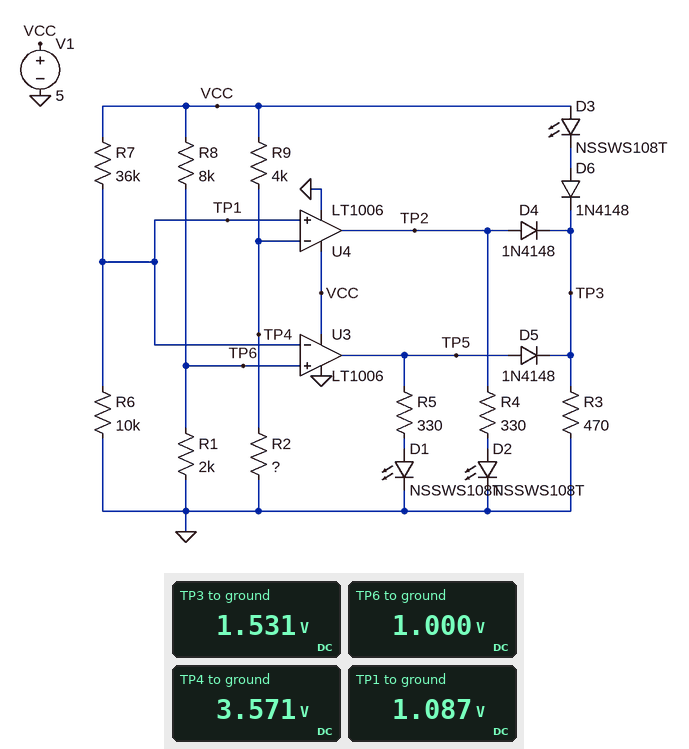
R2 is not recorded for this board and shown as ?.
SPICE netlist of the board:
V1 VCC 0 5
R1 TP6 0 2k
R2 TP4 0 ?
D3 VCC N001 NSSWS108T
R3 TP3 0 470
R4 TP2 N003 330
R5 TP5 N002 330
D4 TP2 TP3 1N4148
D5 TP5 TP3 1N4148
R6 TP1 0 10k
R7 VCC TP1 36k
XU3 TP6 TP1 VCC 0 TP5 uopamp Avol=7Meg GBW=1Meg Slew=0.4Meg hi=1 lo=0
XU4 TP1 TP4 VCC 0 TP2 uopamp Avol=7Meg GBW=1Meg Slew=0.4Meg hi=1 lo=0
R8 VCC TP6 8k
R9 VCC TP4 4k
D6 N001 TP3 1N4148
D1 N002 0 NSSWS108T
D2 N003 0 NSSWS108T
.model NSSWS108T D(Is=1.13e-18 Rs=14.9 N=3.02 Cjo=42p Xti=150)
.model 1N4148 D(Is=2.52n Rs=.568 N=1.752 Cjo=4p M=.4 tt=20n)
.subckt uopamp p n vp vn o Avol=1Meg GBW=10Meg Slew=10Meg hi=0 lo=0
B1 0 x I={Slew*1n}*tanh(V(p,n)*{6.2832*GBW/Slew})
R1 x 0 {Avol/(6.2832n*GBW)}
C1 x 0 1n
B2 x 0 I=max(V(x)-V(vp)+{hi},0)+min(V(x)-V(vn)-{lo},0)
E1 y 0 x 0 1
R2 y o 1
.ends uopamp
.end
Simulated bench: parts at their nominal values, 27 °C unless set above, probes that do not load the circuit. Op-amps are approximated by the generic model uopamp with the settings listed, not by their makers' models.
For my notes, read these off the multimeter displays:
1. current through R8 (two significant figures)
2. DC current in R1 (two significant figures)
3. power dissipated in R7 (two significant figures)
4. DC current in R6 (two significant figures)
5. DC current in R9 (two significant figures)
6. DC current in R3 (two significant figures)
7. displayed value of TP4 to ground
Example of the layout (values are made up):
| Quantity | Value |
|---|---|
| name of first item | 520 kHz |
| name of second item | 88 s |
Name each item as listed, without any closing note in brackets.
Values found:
| Quantity | Value |
|---|---|
| current through R8 | 500 µA |
| DC current in R1 | 500 µA |
| power dissipated in R7 | 430 µW |
| DC current in R6 | 110 µA |
| DC current in R9 | 360 µA |
| DC current in R3 | 3.3 mA |
| displayed value of TP4 to ground | 3.571 V |
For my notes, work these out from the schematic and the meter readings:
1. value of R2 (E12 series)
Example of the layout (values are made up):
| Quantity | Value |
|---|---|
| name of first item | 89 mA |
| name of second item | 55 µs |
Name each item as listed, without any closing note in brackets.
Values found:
| Quantity | Value |
|---|---|
| value of R2 | 10 kΩ |
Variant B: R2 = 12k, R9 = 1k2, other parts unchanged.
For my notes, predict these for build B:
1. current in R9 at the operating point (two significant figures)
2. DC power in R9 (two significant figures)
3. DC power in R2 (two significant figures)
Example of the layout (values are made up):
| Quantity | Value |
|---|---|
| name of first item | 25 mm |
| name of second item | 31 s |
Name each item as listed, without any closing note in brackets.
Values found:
| Quantity | Value |
|---|---|
| current in R9 at the operating point | 380 µA |
| DC power in R9 | 170 µW |
| DC power in R2 | 1.7 mW |
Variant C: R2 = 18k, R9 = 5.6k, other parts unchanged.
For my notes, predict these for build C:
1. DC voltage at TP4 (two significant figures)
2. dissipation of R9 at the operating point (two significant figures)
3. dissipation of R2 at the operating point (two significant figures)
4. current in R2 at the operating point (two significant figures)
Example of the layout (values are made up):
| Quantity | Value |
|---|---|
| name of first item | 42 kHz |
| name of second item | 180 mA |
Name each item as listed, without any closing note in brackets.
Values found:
| Quantity | Value |
|---|---|
| DC voltage at TP4 | 3.8 V |
| dissipation of R9 at the operating point | 250 µW |
| dissipation of R2 at the operating point | 810 µW |
| current in R2 at the operating point | 210 µA |
